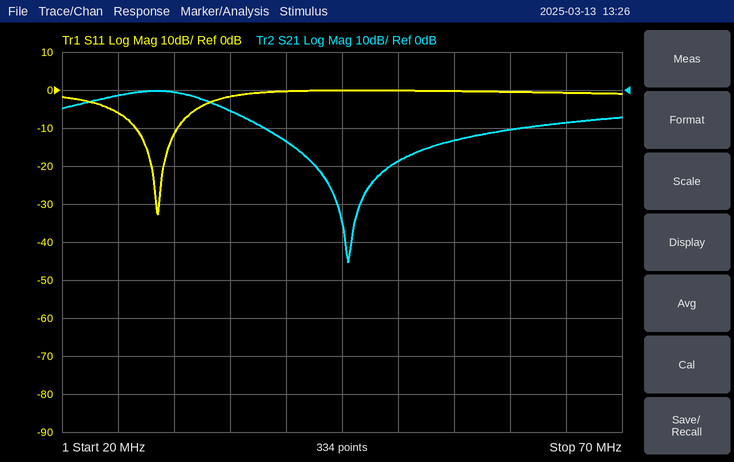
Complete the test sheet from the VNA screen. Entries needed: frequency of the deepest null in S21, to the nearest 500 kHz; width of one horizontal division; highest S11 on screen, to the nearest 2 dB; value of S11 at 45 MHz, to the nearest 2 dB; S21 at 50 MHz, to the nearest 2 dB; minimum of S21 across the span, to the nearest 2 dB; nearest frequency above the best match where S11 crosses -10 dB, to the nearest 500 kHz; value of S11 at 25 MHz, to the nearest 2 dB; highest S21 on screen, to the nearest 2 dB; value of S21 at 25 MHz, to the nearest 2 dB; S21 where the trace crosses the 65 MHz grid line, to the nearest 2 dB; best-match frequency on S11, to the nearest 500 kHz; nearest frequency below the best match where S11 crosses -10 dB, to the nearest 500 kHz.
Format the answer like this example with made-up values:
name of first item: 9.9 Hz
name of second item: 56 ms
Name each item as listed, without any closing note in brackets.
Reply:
frequency of the deepest null in S21, to the nearest 500 kHz: 45.5 MHz
width of one horizontal division: 5 MHz
highest S11 on screen, to the nearest 2 dB: 0 dB
value of S11 at 45 MHz, to the nearest 2 dB: 0 dB
S21 at 50 MHz, to the nearest 2 dB: -18 dB
minimum of S21 across the span, to the nearest 2 dB: -46 dB
nearest frequency above the best match where S11 crosses -10 dB, to the nearest 500 kHz: 30.5 MHz
value of S11 at 25 MHz, to the nearest 2 dB: -6 dB
highest S21 on screen, to the nearest 2 dB: 0 dB
value of S21 at 25 MHz, to the nearest 2 dB: -2 dB
S21 where the trace crosses the 65 MHz grid line, to the nearest 2 dB: -8 dB
best-match frequency on S11, to the nearest 500 kHz: 28.5 MHz
nearest frequency below the best match where S11 crosses -10 dB, to the nearest 500 kHz: 26.5 MHz
